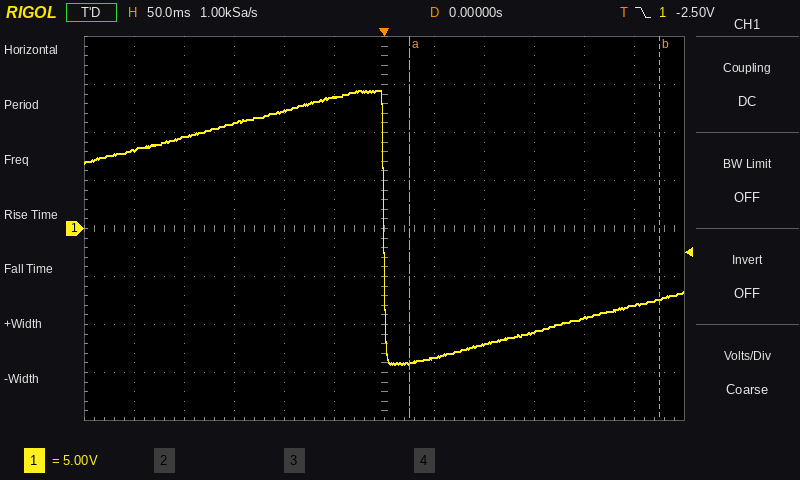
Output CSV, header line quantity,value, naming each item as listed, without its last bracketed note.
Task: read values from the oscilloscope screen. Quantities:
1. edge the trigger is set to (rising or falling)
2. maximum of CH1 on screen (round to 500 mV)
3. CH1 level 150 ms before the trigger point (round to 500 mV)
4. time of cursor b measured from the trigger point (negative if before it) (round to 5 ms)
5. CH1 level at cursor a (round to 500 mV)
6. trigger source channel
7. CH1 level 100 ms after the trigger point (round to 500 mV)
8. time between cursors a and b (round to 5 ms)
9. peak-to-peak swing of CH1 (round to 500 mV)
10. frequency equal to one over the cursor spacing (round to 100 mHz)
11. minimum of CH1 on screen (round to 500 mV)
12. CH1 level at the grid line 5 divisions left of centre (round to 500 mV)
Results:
quantity,value
edge the trigger is set to,falling
maximum of CH1 on screen,14.5 V
CH1 level 150 ms before the trigger point,11.0 V
time of cursor b measured from the trigger point (negative if before it),+275 ms
CH1 level at cursor a,-14.0 V
trigger source channel,CH1
CH1 level 100 ms after the trigger point,-12.0 V
time between cursors a and b,250 ms
peak-to-peak swing of CH1,28.5 V
frequency equal to one over the cursor spacing,4.0 Hz
minimum of CH1 on screen,-14.0 V
CH1 level at the grid line 5 divisions left of centre,8.0 V
